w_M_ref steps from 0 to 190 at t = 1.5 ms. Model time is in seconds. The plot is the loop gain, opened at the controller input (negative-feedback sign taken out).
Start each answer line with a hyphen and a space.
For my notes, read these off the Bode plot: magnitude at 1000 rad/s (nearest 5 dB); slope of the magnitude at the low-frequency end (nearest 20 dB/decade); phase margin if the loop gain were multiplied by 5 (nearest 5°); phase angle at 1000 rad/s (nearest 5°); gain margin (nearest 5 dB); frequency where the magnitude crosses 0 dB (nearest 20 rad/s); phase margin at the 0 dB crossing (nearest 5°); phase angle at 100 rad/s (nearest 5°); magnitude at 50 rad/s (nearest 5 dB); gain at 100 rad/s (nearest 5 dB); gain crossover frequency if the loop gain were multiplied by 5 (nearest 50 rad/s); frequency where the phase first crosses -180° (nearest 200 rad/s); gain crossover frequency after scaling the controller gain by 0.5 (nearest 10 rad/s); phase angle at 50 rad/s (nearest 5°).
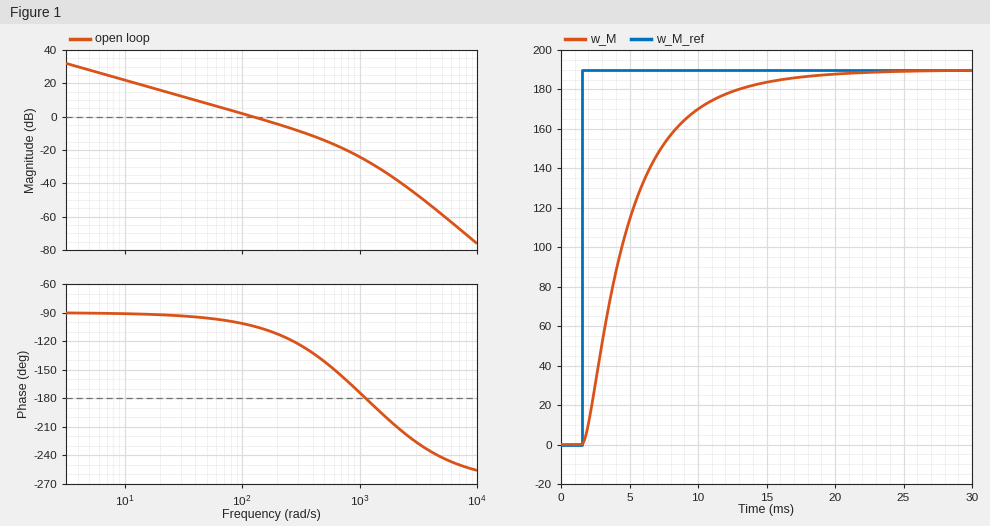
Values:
- -25 dB
- -20 dB/decade
- 40°
- -175°
- 25 dB
- 120 rad/s
- 75°
- -100°
- 10 dB
- 0 dB
- 500 rad/s
- 1200 rad/s
- 60 rad/s
- -95°
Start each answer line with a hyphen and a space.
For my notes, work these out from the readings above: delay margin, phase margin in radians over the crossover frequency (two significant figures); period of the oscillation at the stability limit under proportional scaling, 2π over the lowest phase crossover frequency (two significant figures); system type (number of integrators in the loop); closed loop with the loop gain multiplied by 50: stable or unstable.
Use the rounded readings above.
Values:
- 0.011 s
- 0.0052 s
- 1
- unstable
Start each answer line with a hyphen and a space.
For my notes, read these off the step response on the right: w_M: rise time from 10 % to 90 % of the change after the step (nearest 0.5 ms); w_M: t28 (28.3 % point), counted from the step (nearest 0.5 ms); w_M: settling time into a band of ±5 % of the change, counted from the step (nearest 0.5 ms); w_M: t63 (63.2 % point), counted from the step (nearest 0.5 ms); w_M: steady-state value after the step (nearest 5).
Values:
- 8.0 ms
- 1.5 ms
- 11.5 ms
- 4.0 ms
- 190
